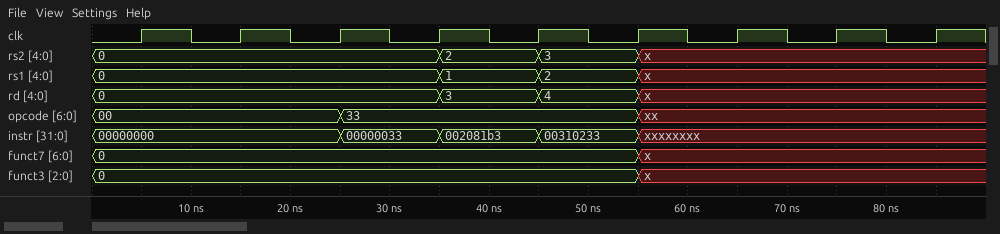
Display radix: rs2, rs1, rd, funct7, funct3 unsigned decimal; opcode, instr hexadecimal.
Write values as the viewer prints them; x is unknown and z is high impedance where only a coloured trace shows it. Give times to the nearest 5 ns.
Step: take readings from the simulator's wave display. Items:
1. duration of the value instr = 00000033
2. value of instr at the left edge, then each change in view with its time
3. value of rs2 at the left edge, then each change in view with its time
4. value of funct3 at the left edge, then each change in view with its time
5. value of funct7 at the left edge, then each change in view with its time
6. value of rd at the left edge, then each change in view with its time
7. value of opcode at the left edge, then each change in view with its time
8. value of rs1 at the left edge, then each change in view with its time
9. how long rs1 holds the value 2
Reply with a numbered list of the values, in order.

1. 10 ns
2. 00000000, 00000033 at 25 ns, 002081b3 at 35 ns, 00310233 at 45 ns, xxxxxxxx at 55 ns
3. 0, 2 at 35 ns, 3 at 45 ns, x at 55 ns
4. 0, x at 55 ns
5. 0, x at 55 ns
6. 0, 3 at 35 ns, 4 at 45 ns, x at 55 ns
7. 00, 33 at 25 ns, xx at 55 ns
8. 0, 1 at 35 ns, 2 at 45 ns, x at 55 ns
9. 10 ns
